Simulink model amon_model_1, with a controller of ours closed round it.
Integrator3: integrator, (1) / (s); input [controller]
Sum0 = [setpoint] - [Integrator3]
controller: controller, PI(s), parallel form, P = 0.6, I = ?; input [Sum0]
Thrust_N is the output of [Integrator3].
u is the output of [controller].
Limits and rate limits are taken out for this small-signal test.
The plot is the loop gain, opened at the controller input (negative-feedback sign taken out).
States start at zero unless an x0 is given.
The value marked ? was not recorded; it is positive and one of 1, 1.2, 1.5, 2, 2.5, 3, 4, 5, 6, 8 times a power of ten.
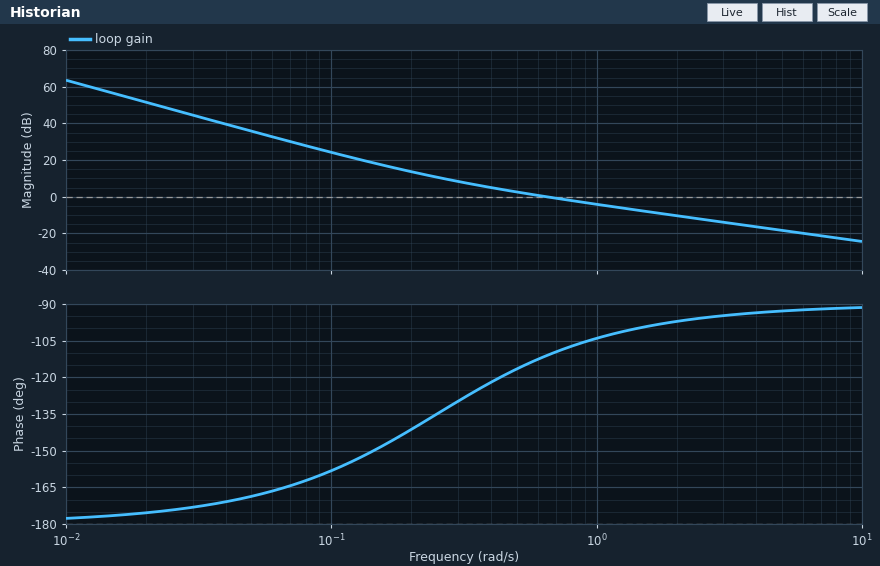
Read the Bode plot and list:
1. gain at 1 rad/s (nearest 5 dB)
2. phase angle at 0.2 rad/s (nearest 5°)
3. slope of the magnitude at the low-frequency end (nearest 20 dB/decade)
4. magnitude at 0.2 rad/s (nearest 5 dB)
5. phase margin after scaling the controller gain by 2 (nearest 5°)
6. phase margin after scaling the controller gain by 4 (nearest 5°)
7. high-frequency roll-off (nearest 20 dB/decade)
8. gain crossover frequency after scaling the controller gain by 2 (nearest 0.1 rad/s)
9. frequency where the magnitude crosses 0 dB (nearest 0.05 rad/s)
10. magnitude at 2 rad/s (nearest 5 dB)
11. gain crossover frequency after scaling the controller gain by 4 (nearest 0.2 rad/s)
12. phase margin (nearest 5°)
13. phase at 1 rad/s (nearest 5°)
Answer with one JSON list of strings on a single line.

["-5 dB", "-140°", "-40 dB/decade", "15 dB", "80°", "85°", "-20 dB/decade", "1.2 rad/s", "0.65 rad/s", "-10 dB", "2.4 rad/s", "70°", "-105°"]
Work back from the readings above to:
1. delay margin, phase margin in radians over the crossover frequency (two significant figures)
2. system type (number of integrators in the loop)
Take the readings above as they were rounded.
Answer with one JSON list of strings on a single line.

["1.9 s", "2"]
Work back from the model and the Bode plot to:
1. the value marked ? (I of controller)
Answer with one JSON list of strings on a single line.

["0.15"]
